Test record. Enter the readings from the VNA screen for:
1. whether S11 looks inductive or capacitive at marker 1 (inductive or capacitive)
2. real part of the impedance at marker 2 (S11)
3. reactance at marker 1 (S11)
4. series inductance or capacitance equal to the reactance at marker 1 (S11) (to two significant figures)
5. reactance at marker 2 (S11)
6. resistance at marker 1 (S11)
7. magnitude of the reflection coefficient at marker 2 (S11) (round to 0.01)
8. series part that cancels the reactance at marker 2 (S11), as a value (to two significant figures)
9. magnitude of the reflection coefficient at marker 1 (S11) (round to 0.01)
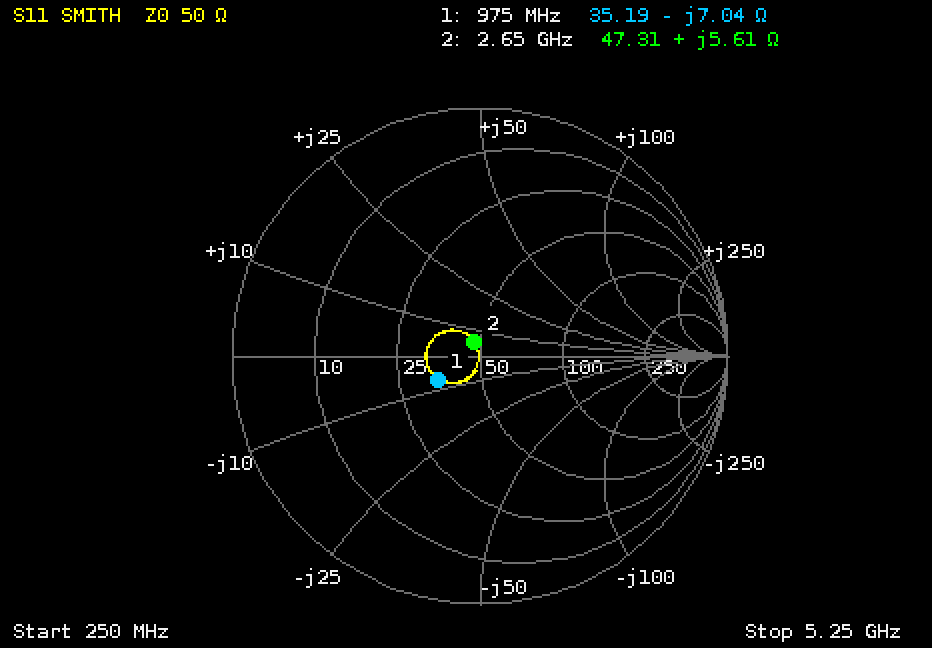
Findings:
capacitive
47.31 Ω
-7.04 Ω
23 pF
+5.61 Ω
35.19 Ω
0.06
11 pF
0.19
